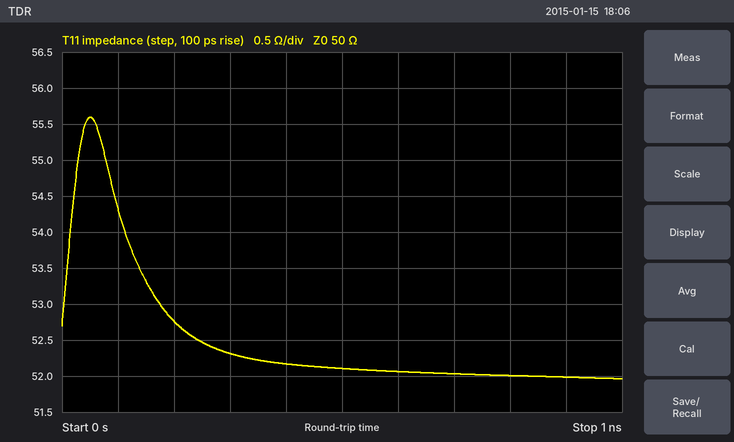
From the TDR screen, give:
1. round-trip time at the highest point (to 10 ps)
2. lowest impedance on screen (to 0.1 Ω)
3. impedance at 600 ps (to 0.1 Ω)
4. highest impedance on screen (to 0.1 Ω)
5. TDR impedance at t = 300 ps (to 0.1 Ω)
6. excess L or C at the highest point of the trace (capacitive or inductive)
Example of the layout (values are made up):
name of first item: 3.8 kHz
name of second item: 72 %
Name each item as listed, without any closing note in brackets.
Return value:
round-trip time at the highest point: 50 ps
lowest impedance on screen: 52.0 Ω
impedance at 600 ps: 52.1 Ω
highest impedance on screen: 55.6 Ω
TDR impedance at t = 300 ps: 52.3 Ω
excess L or C at the highest point of the trace: inductive
